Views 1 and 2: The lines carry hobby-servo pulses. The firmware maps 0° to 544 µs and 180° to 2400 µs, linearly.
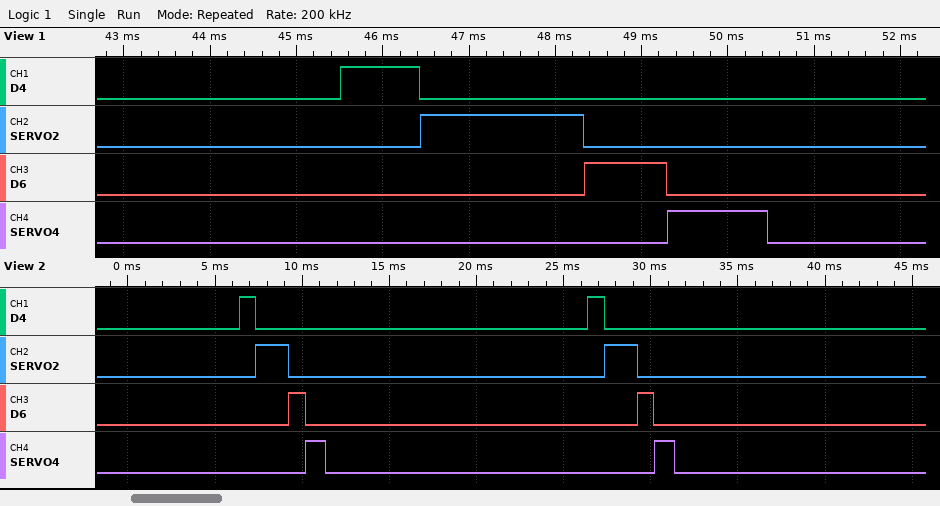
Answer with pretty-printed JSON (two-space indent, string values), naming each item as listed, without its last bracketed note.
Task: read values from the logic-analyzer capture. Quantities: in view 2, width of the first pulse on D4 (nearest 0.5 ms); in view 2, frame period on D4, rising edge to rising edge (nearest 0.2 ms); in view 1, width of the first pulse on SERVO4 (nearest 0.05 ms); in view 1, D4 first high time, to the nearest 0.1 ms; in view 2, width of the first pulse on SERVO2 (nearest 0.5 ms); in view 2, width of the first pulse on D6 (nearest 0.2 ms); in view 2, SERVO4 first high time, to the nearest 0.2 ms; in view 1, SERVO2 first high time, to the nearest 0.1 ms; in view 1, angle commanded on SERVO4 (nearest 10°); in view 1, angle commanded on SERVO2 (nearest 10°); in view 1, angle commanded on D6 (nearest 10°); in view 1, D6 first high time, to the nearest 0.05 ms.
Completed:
{
  "in view 2, width of the first pulse on D4": "1.0 ms",
  "in view 2, frame period on D4, rising edge to rising edge": "20.0 ms",
  "in view 1, width of the first pulse on SERVO4": "1.15 ms",
  "in view 1, D4 first high time, to the nearest 0.1 ms": "0.9 ms",
  "in view 2, width of the first pulse on SERVO2": "2.0 ms",
  "in view 2, width of the first pulse on D6": "1.0 ms",
  "in view 2, SERVO4 first high time, to the nearest 0.2 ms": "1.2 ms",
  "in view 1, SERVO2 first high time, to the nearest 0.1 ms": "1.9 ms",
  "in view 1, angle commanded on SERVO4": "60°",
  "in view 1, angle commanded on SERVO2": "130°",
  "in view 1, angle commanded on D6": "40°",
  "in view 1, D6 first high time, to the nearest 0.05 ms": "0.95 ms"
}
